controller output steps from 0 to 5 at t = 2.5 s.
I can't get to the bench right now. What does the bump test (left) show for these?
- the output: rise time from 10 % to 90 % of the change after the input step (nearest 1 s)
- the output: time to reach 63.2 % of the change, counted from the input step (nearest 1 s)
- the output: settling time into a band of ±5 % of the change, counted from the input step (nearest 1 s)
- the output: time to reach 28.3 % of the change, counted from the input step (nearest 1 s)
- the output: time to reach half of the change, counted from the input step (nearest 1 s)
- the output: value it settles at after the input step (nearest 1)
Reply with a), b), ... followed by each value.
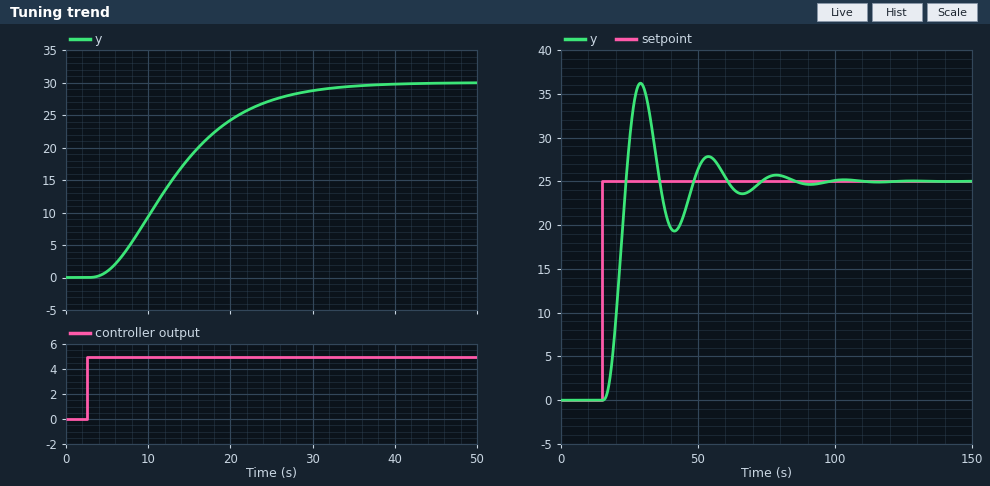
a) 18 s
b) 13 s
c) 26 s
d) 7 s
e) 10 s
f) 30
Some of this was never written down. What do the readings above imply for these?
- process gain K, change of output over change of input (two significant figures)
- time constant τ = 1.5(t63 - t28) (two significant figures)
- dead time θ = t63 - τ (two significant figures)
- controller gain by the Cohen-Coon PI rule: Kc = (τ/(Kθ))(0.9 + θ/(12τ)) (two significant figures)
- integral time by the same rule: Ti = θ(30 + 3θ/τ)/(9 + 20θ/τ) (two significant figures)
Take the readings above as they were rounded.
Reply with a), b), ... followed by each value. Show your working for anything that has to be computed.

a) (30 - 0) / 5 = 6.0
b) 1.5 × (13 - 7) = 9.0 s
c) 13 - 9 = 4.0 s
d) 9 / (6 × 4) × (0.9 + 4 / (12 × 9)) = 0.35
e) 4 × (30 + 3 × 4 / 9) / (9 + 20 × 4 / 9) = 7.0 s
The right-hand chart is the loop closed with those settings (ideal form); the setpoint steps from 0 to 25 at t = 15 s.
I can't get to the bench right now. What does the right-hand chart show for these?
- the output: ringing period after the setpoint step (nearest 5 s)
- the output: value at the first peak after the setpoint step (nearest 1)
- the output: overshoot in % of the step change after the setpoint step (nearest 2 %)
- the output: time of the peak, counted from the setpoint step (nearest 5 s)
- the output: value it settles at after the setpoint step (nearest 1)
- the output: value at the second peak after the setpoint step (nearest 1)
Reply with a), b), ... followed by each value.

a) 25 s
b) 36
c) 44 %
d) 15 s
e) 25
f) 28
